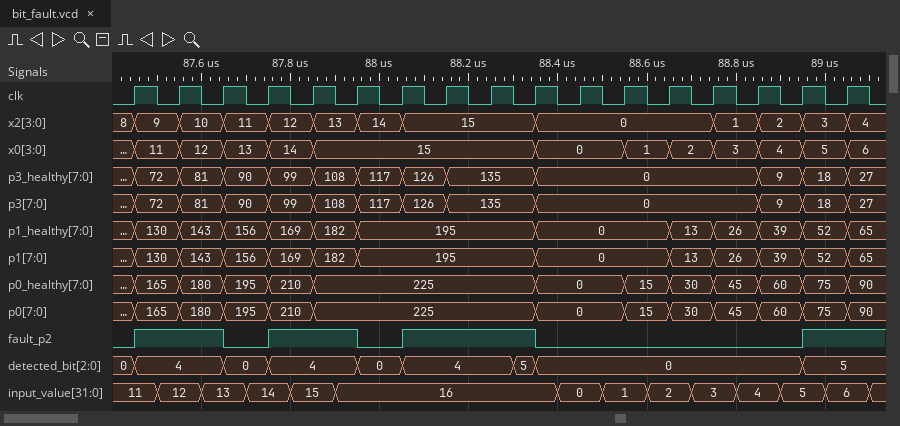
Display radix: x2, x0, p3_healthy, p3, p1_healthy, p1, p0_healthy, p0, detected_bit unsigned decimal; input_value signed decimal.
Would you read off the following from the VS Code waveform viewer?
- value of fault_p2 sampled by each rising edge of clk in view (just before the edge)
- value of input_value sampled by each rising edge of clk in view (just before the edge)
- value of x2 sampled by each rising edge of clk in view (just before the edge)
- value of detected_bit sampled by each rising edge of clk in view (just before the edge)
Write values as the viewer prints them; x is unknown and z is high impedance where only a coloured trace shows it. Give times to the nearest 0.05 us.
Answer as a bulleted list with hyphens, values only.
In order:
- 0 1 1 0 1 1 0 1 1 1 0 0 0 0 0 0 1
- 11, 12, 13, 14, 15, 16, 16, 16, 16, 16, 0, 1, 2, 3, 4, 5, 6
- 8, 9, 10, 11, 12, 13, 14, 15, 15, 15, 0, 0, 0, 0, 1, 2, 3
- 0, 4, 4, 0, 4, 4, 0, 4, 4, 5, 0, 0, 0, 0, 0, 0, 5
